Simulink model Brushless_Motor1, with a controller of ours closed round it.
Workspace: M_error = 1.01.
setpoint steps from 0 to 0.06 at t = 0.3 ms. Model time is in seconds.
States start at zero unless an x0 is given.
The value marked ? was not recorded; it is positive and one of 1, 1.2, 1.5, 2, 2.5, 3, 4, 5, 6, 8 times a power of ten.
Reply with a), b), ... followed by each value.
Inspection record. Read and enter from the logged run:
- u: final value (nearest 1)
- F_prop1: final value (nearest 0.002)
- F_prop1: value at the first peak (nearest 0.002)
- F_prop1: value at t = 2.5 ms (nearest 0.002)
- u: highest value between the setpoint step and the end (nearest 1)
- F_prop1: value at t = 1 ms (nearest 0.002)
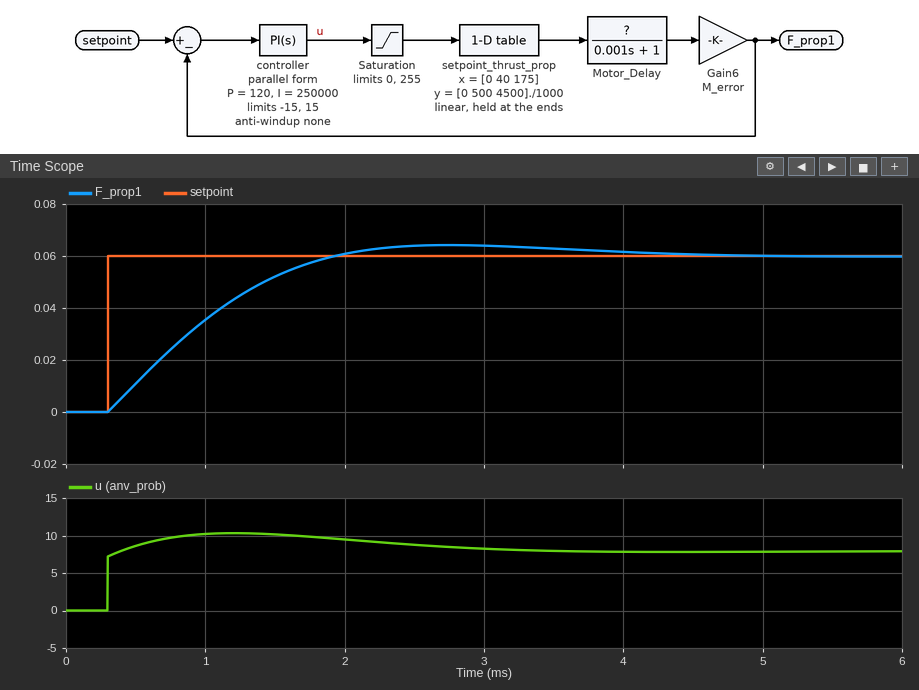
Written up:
a) 8
b) 0.060
c) 0.064
d) 0.064
e) 10
f) 0.036
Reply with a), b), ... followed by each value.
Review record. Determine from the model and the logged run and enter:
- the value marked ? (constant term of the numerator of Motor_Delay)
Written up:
a) 0.6
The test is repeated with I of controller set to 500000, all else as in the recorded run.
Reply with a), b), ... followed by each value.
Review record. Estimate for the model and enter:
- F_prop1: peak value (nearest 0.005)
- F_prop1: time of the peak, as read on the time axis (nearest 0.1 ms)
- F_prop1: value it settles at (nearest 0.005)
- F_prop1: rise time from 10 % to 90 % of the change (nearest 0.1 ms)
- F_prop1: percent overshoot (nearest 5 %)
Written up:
a) 0.070
b) 1.9 ms
c) 0.060
d) 0.7 ms
e) 20 %
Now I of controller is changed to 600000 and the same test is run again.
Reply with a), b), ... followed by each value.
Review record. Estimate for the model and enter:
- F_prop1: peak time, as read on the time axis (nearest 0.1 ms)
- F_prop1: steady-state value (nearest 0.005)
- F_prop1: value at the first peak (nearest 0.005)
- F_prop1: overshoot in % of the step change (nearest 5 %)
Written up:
a) 1.7 ms
b) 0.060
c) 0.075
d) 25 %
